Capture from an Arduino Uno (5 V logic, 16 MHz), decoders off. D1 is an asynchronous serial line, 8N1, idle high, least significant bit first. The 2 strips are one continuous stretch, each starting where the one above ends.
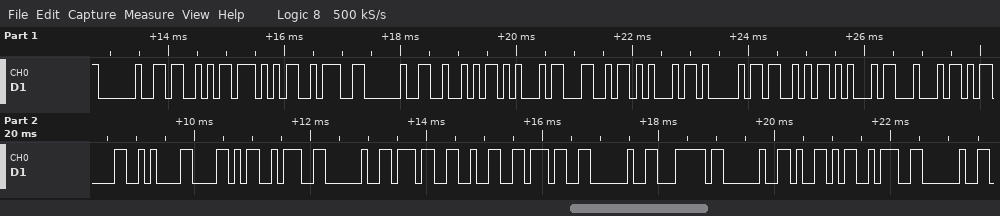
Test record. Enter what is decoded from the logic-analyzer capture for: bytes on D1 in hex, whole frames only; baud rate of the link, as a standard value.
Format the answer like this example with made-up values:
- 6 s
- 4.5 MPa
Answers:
- 20 53 57 3A 20 52 45 4C 45 41 53 45 44 0D 0A 58 3A 20 37 32 37 20 7C 20 59 3A 20
- 9600 baud
